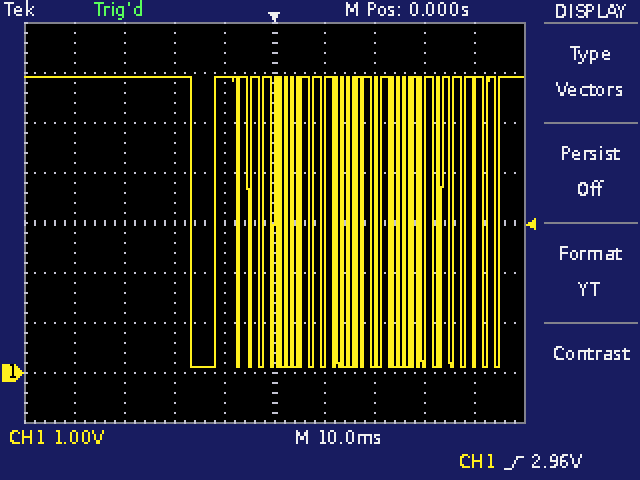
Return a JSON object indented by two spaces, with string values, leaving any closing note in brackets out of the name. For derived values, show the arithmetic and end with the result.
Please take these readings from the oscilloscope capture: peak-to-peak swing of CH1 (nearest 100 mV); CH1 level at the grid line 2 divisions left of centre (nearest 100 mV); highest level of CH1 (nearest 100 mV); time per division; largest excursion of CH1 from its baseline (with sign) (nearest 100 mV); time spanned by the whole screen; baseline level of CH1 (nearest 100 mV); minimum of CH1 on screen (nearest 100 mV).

{
  "peak-to-peak swing of CH1": "5.9 V − (100 mV) = 5.8 V",
  "CH1 level at the grid line 2 divisions left of centre": "5.9 V",
  "highest level of CH1": "5.9 V",
  "time per division": "10 ms",
  "largest excursion of CH1 from its baseline (with sign)": "100 mV − (5.9 V) = -5.8 V",
  "time spanned by the whole screen": "100 ms",
  "baseline level of CH1": "5.9 V",
  "minimum of CH1 on screen": "100 mV"
}
